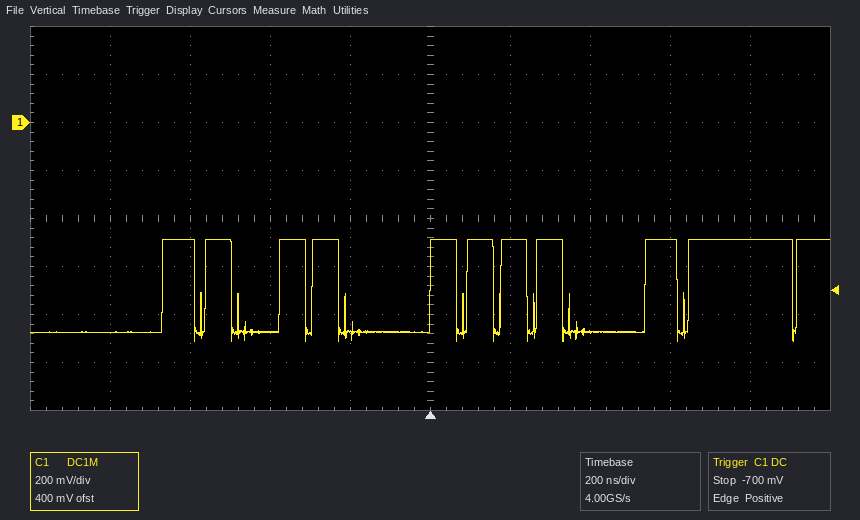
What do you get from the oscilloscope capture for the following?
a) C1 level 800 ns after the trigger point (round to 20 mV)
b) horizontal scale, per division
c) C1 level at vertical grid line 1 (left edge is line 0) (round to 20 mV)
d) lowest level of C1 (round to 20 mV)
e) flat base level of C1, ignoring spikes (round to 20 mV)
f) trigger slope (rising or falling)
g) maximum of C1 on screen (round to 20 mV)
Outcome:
-480 mV
200 ns
-880 mV
-920 mV
-880 mV
rising
-480 mV
